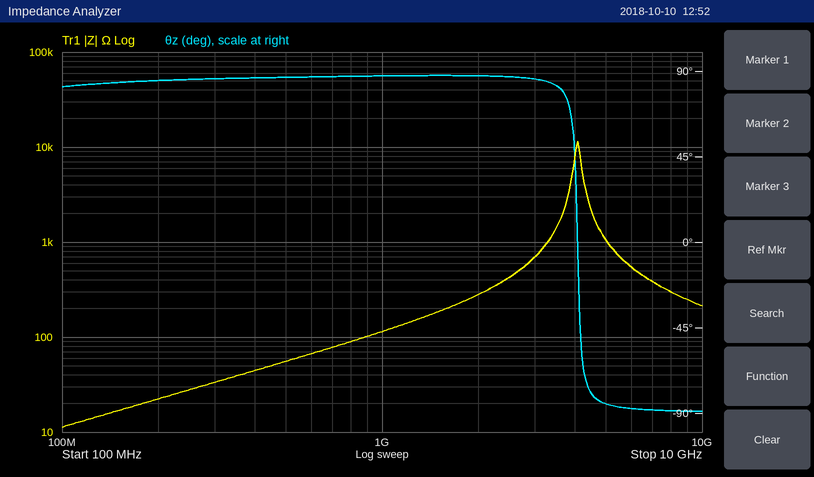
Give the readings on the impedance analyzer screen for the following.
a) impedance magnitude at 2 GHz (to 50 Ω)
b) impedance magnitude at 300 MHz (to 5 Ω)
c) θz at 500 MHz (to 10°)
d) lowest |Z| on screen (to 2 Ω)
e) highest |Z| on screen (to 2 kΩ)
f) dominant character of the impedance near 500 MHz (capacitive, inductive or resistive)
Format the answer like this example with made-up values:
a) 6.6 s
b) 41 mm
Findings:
a) 300 Ω
b) 35 Ω
c) 90°
d) 12 Ω
e) 12 kΩ
f) inductive
